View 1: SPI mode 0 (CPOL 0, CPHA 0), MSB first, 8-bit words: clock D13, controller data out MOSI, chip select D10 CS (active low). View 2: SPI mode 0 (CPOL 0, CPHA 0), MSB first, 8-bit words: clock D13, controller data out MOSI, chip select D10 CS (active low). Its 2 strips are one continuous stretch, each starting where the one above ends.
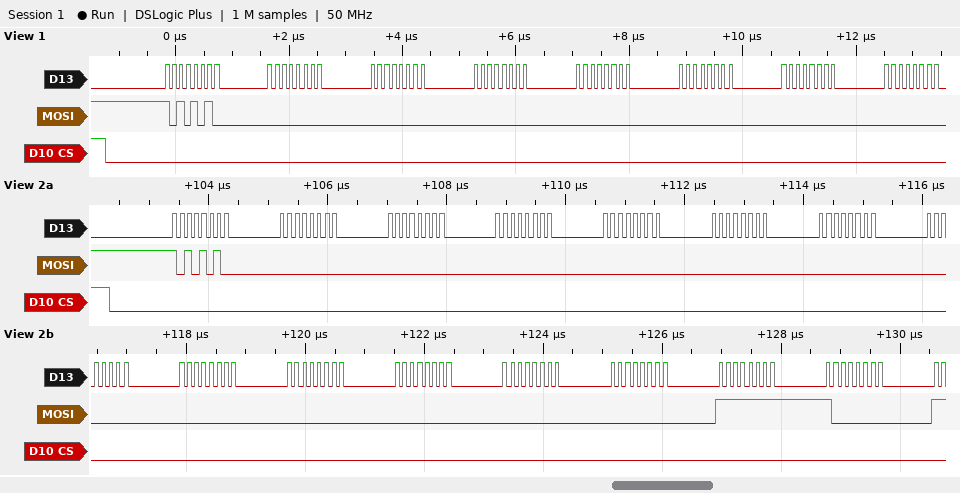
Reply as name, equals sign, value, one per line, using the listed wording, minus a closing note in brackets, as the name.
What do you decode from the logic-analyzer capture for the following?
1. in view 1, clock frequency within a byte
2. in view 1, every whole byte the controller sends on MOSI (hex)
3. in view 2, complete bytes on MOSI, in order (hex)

in view 1, clock frequency within a byte = 8 MHz
in view 1, every whole byte the controller sends on MOSI = 0xAA 0x00 0x00 0x00 0x00 0x00 0x00 0x00
in view 2, complete bytes on MOSI, in order = AA 00 00 00 00 00 00 00 00 00 00 00 00 FF 80
